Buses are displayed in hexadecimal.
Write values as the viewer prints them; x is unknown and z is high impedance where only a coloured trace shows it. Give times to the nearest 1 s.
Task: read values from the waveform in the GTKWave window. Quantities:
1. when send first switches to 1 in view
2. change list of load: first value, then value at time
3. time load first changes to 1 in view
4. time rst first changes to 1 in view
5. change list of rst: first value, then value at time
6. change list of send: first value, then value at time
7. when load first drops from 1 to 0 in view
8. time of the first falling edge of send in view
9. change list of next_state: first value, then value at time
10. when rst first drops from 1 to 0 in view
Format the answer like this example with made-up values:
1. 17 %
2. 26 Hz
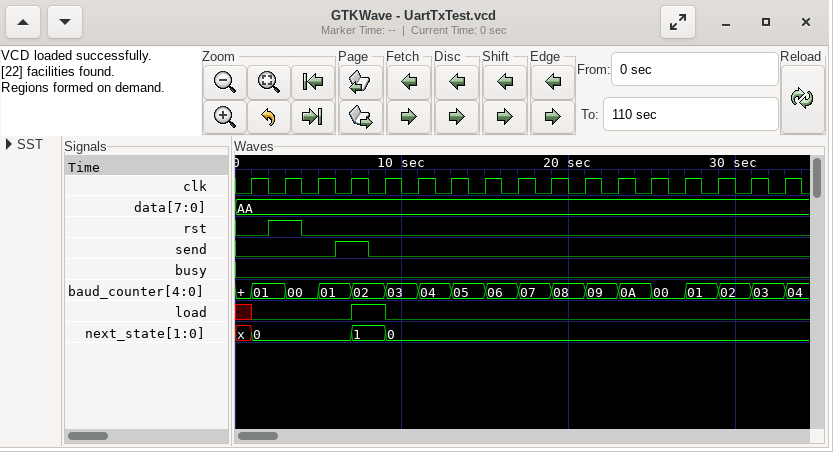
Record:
1. 6 s
2. x, 0 at 1 s, 1 at 7 s, 0 at 9 s
3. 7 s
4. 2 s
5. 0, 1 at 2 s, 0 at 4 s
6. 0, 1 at 6 s, 0 at 8 s
7. 9 s
8. 8 s
9. x, 0 at 1 s, 1 at 7 s, 0 at 9 s
10. 4 s
